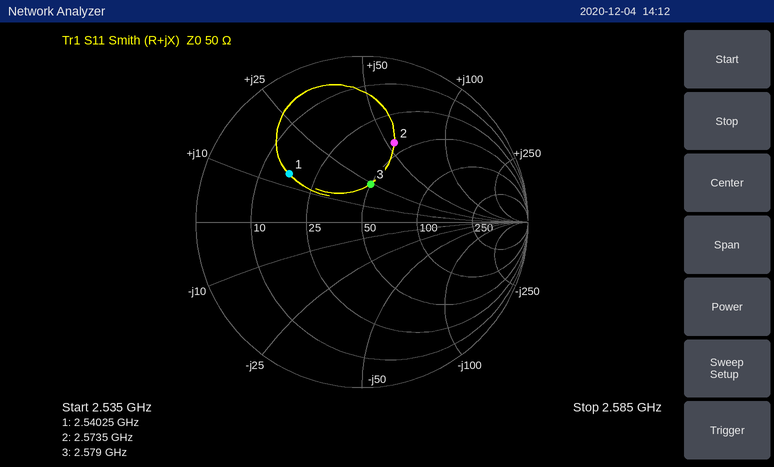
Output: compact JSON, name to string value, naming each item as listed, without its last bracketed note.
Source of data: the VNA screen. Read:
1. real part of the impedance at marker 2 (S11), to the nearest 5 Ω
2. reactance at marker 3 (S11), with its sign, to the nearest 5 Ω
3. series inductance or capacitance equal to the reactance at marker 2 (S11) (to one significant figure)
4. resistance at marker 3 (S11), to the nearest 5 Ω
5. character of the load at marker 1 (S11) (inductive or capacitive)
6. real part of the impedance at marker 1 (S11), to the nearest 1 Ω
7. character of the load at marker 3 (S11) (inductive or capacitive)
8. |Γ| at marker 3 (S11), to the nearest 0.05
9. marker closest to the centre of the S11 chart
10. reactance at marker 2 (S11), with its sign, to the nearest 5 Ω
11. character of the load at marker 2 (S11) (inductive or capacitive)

{"real part of the impedance at marker 2 (S11), to the nearest 5 Ω": "40 Ω", "reactance at marker 3 (S11), with its sign, to the nearest 5 Ω": "+25 Ω", "series inductance or capacitance equal to the reactance at marker 2 (S11)": "3 nH", "resistance at marker 3 (S11), to the nearest 5 Ω": "50 Ω", "character of the load at marker 1 (S11)": "inductive", "real part of the impedance at marker 1 (S11), to the nearest 1 Ω": "17 Ω", "character of the load at marker 3 (S11)": "inductive", "|Γ| at marker 3 (S11), to the nearest 0.05": "0.25", "marker closest to the centre of the S11 chart": "marker 3", "reactance at marker 2 (S11), with its sign, to the nearest 5 Ω": "+55 Ω", "character of the load at marker 2 (S11)": "inductive"}
